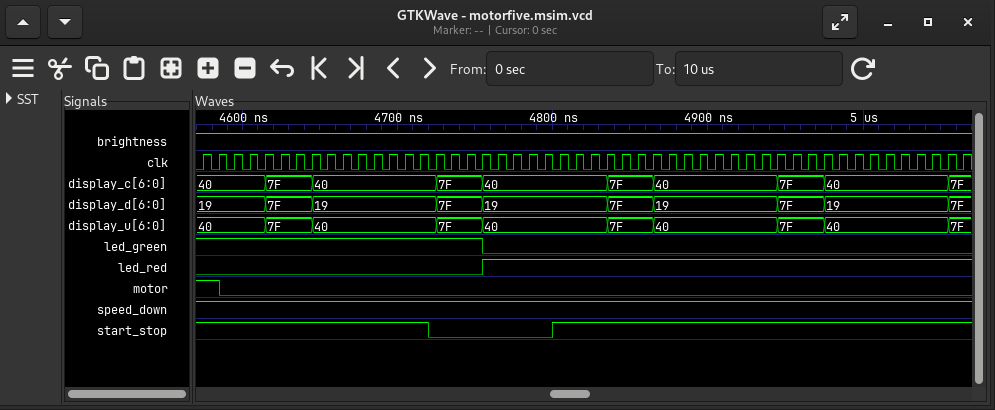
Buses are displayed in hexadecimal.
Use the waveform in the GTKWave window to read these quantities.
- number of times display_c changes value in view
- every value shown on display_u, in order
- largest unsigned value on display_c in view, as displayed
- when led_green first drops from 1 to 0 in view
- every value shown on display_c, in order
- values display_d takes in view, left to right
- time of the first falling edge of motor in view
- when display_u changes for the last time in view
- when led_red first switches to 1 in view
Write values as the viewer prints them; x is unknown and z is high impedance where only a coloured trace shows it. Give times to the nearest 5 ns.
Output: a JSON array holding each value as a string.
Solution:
["9", "40, 7F, 40, 7F, 40, 7F, 40, 7F, 40, 7F", "7F", "4755 ns", "40, 7F, 40, 7F, 40, 7F, 40, 7F, 40, 7F", "19, 7F, 19, 7F, 19, 7F, 19, 7F, 19, 7F", "4585 ns", "5055 ns", "4755 ns"]
